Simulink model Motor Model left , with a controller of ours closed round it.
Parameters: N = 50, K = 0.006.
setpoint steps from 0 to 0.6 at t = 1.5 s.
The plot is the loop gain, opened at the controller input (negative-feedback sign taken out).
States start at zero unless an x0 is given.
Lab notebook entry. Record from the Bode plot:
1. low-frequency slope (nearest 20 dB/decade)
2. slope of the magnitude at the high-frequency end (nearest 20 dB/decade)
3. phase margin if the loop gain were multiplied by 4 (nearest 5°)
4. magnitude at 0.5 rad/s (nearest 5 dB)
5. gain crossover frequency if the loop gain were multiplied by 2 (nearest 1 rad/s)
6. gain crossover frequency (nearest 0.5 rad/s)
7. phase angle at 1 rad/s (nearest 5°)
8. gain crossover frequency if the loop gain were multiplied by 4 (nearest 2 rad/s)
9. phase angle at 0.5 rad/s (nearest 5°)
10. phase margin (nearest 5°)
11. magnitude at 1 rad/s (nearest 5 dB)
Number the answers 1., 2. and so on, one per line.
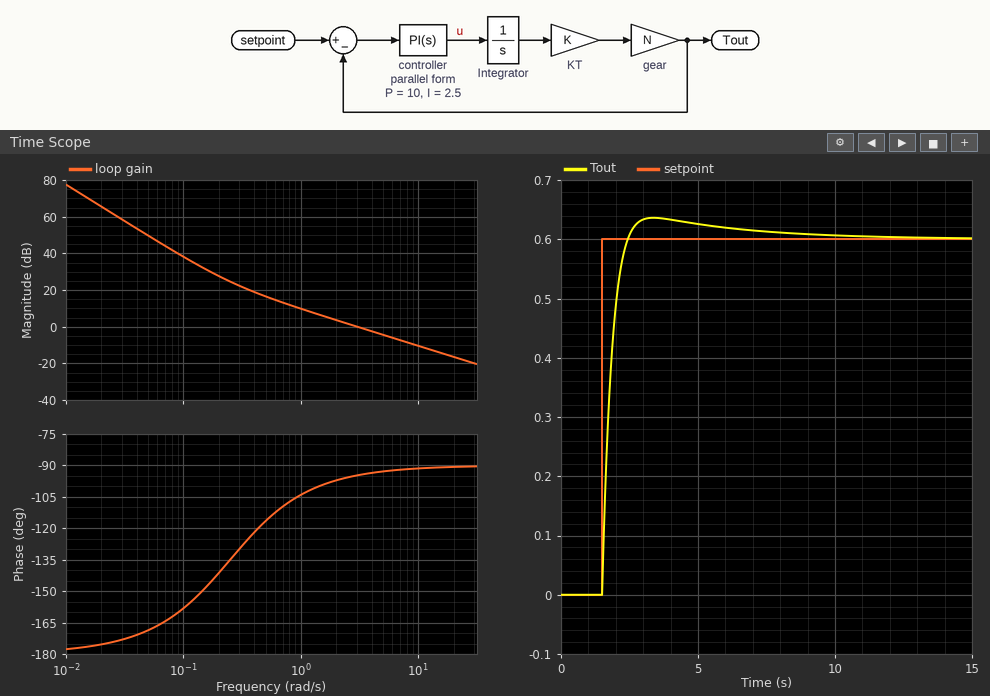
1. -40 dB/decade
2. -20 dB/decade
3. 90°
4. 15 dB
5. 6 rad/s
6. 3.0 rad/s
7. -105°
8. 12 rad/s
9. -115°
10. 85°
11. 10 dB
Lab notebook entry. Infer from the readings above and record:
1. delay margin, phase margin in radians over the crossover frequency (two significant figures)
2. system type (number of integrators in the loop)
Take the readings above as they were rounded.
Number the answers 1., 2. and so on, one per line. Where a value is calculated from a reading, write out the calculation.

1. 85 × π / 180 / 3 = 0.49 s
2. 2
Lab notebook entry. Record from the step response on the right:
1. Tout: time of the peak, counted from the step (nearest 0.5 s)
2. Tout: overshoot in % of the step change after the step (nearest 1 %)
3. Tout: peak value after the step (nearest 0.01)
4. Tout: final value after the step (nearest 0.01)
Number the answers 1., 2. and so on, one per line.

1. 2.0 s
2. 6 %
3. 0.64
4. 0.60
